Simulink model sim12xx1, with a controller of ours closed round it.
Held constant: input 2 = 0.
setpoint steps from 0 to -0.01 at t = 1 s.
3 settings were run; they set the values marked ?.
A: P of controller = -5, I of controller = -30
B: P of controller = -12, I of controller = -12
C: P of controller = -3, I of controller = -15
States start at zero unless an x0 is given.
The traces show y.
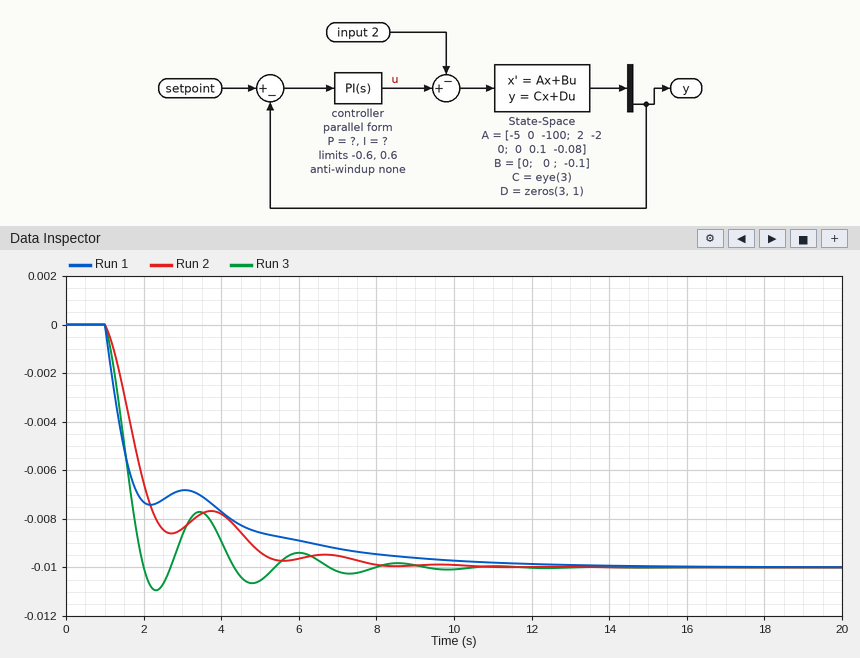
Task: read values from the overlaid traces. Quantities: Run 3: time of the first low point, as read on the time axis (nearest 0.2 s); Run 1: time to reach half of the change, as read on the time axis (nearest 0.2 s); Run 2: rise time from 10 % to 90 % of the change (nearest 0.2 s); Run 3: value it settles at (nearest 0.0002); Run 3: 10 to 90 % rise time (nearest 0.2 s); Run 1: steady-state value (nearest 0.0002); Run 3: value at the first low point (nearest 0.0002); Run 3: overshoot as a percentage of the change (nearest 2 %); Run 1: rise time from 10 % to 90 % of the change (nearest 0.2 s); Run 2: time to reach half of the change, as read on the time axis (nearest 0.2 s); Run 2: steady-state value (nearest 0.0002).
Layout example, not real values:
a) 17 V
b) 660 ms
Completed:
a) 2.4 s
b) 1.4 s
c) 3.6 s
d) -0.0100
e) 0.8 s
f) -0.0100
g) -0.0110
h) 10 %
i) 5.2 s
j) 1.8 s
k) -0.0100
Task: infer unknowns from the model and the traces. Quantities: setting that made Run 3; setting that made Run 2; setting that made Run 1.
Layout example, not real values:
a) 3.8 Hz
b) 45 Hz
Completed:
a) A
b) C
c) B
